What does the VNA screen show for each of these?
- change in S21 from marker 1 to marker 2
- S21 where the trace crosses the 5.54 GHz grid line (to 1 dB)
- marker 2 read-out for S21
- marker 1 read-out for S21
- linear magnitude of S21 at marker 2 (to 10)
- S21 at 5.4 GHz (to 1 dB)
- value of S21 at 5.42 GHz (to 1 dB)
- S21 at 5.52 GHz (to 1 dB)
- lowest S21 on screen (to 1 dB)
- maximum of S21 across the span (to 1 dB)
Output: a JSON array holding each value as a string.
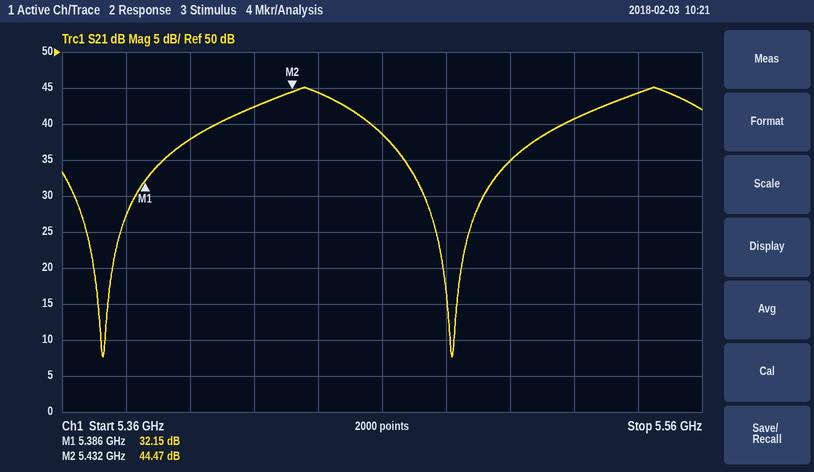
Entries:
["12.32 dB", "44 dB", "44.47 dB", "32.15 dB", "170", "38 dB", "42 dB", "41 dB", "8 dB", "45 dB"]
